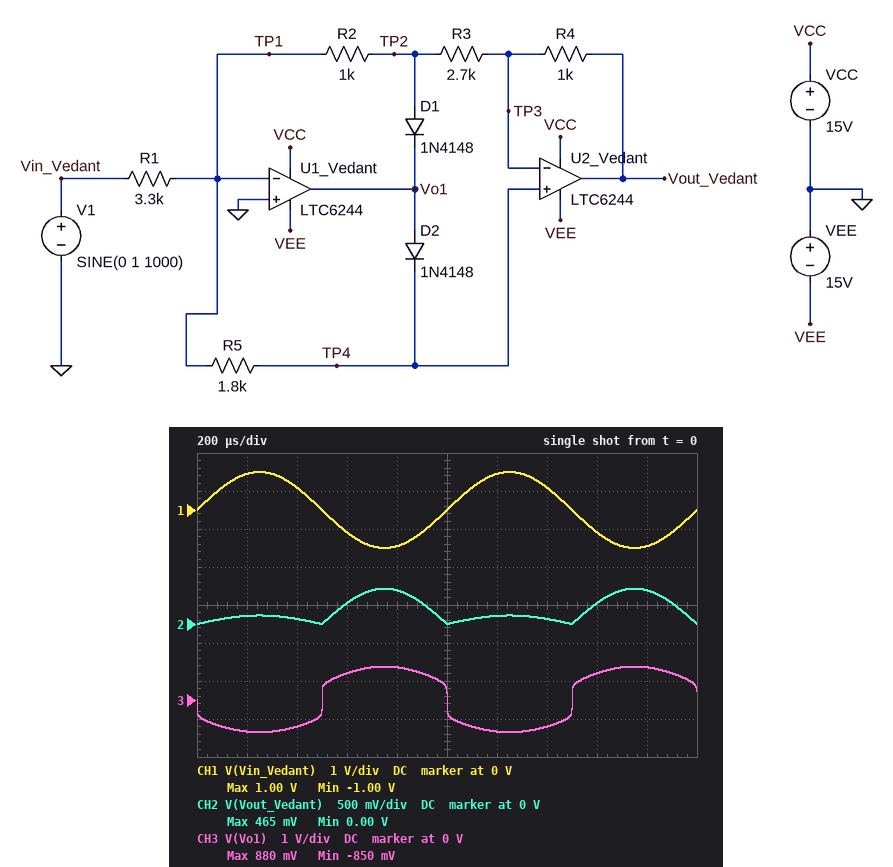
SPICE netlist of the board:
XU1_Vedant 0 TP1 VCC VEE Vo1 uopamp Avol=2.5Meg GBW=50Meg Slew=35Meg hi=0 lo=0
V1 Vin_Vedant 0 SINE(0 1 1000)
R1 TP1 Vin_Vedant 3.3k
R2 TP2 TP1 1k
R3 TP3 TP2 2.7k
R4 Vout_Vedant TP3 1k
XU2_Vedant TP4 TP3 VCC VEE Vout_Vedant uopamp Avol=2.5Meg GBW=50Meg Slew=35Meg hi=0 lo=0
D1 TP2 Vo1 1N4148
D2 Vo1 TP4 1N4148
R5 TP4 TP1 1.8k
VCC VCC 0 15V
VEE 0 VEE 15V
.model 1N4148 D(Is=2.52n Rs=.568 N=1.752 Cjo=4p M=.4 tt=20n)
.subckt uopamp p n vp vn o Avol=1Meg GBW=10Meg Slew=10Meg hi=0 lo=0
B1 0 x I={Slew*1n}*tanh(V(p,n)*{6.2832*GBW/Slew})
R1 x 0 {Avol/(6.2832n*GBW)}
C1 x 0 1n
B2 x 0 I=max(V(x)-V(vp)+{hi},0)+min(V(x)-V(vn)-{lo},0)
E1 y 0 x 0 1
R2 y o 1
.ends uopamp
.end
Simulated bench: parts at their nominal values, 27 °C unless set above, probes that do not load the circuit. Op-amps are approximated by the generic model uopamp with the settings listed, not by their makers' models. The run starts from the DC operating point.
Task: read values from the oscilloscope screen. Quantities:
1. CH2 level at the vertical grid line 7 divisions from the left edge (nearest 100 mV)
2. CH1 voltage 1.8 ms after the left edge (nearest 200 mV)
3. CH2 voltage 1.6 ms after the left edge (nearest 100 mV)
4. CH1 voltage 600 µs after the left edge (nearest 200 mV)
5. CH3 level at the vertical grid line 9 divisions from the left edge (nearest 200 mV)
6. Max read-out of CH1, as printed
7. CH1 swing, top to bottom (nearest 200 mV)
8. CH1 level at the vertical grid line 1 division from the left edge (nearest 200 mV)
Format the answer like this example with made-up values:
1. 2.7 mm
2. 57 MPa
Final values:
1. 100 mV
2. -1.0 V
3. 300 mV
4. -600 mV
5. 800 mV
6. 1.00 V
7. 2.0 V
8. 1.0 V
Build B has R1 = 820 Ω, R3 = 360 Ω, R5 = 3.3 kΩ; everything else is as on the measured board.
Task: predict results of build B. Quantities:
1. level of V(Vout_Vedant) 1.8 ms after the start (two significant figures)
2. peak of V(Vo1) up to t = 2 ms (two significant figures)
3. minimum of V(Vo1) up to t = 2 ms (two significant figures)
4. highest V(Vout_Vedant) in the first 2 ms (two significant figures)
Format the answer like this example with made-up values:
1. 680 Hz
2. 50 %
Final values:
1. 1.9 V
2. 1.7 V
3. -1.9 V
4. 3.4 V
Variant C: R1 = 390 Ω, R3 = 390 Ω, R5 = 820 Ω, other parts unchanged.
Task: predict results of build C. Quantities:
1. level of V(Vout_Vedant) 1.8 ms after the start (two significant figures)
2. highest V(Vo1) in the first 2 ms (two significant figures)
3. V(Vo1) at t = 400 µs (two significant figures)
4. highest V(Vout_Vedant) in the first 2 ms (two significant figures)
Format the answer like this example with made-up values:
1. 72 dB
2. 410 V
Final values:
1. 2.2 V
2. 1.9 V
3. -2.2 V
4. 6.6 V
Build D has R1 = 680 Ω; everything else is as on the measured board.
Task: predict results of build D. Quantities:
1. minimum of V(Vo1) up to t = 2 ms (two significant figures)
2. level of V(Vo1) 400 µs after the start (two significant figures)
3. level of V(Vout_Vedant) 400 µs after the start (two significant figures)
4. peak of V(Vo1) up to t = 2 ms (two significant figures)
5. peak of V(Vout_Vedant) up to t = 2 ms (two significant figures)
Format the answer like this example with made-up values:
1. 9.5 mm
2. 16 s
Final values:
1. -2.1 V
2. -1.5 V
3. 320 mV
4. 2.4 V
5. 2.3 V
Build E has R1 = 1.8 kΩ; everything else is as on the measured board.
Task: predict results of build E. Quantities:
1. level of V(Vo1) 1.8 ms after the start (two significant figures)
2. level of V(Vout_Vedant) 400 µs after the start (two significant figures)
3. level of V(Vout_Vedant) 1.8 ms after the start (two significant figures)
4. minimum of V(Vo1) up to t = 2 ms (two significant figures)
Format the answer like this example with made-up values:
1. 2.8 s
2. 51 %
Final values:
1. 1.2 V
2. 120 mV
3. 810 mV
4. -1.1 V
